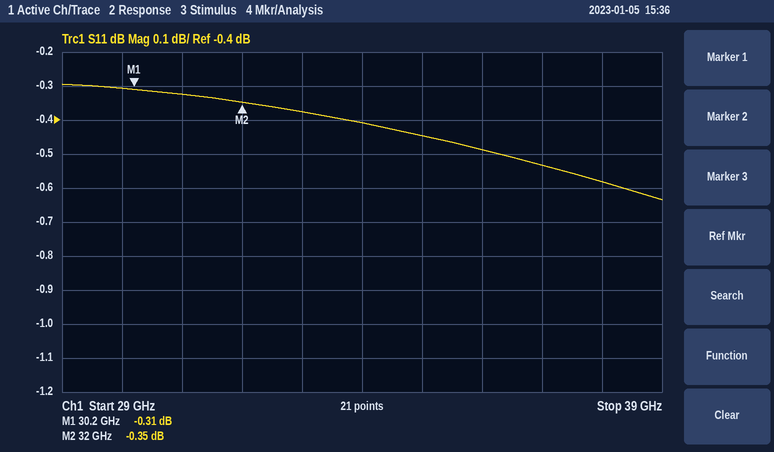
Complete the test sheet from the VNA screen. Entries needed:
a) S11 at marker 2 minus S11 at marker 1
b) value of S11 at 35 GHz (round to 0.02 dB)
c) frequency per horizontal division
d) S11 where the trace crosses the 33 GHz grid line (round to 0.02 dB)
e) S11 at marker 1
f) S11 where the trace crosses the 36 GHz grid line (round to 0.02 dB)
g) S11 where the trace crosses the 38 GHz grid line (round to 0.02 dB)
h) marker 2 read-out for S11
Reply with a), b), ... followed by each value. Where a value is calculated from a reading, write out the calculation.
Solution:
a) -0.35 − (-0.31) = -0.04 dB
b) -0.44 dB
c) 1 GHz
d) -0.38 dB
e) -0.31 dB
f) -0.48 dB
g) -0.58 dB
h) -0.35 dB
